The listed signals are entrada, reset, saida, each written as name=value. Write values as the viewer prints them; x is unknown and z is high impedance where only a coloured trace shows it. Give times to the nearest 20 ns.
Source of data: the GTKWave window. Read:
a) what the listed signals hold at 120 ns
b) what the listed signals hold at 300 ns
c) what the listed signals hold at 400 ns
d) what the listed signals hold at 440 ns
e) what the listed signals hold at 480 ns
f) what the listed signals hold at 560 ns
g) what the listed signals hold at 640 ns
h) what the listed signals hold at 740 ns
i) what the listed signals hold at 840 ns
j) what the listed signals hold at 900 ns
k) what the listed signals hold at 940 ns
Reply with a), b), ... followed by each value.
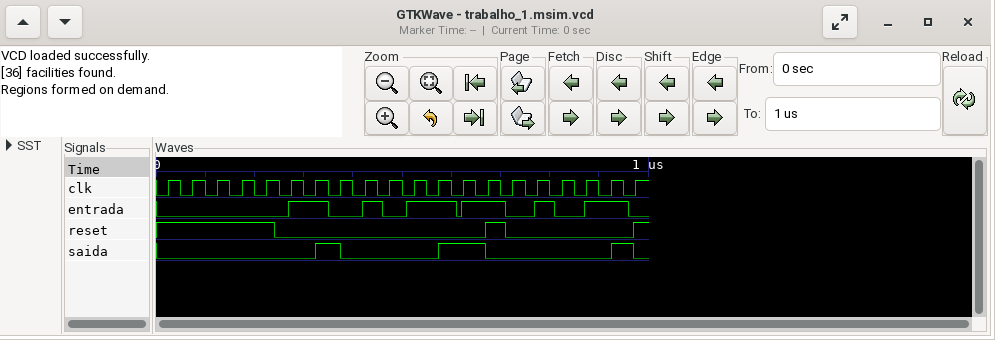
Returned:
a) entrada=0, reset=1, saida=0
b) entrada=1, reset=0, saida=0
c) entrada=0, reset=0, saida=0
d) entrada=1, reset=0, saida=0
e) entrada=0, reset=0, saida=0
f) entrada=1, reset=0, saida=0
g) entrada=1, reset=0, saida=1
h) entrada=0, reset=0, saida=0
i) entrada=0, reset=0, saida=0
j) entrada=1, reset=0, saida=0
k) entrada=1, reset=0, saida=1
